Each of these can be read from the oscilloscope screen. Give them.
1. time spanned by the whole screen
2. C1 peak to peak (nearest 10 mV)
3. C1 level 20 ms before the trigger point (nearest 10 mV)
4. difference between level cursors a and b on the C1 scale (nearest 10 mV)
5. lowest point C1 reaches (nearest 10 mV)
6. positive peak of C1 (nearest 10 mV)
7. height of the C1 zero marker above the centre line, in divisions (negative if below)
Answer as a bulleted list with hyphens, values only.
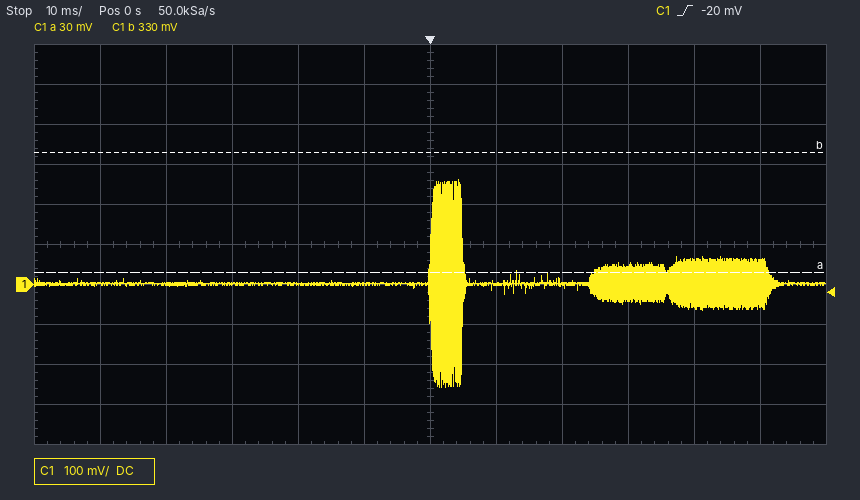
- 120 ms
- 520 mV
- 0 mV
- 300 mV
- -260 mV
- 260 mV
- -1.0 div
